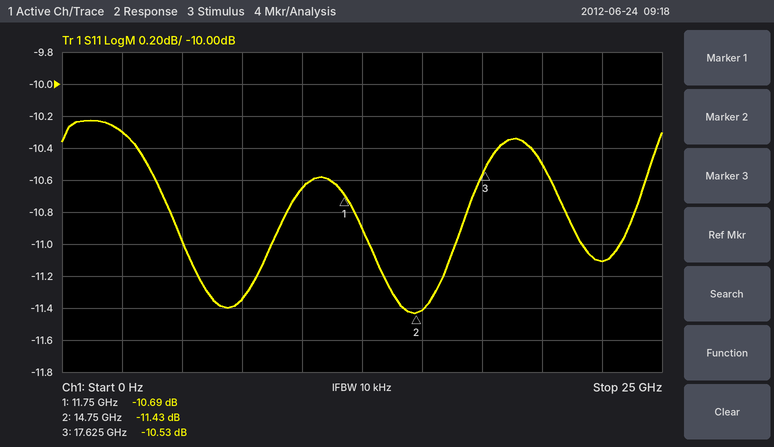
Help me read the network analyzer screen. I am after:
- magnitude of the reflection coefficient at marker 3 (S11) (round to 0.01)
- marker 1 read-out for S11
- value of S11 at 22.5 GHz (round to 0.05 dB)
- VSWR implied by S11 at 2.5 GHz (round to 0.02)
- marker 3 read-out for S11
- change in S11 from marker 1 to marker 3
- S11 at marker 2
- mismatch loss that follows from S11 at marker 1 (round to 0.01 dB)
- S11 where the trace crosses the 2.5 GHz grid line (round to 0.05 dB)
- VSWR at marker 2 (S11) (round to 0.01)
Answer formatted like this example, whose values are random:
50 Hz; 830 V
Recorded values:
0.30; -10.69 dB; -11.10 dB; 1.88; -10.53 dB; 0.16 dB; -11.43 dB; 0.39 dB; -10.30 dB; 1.73
